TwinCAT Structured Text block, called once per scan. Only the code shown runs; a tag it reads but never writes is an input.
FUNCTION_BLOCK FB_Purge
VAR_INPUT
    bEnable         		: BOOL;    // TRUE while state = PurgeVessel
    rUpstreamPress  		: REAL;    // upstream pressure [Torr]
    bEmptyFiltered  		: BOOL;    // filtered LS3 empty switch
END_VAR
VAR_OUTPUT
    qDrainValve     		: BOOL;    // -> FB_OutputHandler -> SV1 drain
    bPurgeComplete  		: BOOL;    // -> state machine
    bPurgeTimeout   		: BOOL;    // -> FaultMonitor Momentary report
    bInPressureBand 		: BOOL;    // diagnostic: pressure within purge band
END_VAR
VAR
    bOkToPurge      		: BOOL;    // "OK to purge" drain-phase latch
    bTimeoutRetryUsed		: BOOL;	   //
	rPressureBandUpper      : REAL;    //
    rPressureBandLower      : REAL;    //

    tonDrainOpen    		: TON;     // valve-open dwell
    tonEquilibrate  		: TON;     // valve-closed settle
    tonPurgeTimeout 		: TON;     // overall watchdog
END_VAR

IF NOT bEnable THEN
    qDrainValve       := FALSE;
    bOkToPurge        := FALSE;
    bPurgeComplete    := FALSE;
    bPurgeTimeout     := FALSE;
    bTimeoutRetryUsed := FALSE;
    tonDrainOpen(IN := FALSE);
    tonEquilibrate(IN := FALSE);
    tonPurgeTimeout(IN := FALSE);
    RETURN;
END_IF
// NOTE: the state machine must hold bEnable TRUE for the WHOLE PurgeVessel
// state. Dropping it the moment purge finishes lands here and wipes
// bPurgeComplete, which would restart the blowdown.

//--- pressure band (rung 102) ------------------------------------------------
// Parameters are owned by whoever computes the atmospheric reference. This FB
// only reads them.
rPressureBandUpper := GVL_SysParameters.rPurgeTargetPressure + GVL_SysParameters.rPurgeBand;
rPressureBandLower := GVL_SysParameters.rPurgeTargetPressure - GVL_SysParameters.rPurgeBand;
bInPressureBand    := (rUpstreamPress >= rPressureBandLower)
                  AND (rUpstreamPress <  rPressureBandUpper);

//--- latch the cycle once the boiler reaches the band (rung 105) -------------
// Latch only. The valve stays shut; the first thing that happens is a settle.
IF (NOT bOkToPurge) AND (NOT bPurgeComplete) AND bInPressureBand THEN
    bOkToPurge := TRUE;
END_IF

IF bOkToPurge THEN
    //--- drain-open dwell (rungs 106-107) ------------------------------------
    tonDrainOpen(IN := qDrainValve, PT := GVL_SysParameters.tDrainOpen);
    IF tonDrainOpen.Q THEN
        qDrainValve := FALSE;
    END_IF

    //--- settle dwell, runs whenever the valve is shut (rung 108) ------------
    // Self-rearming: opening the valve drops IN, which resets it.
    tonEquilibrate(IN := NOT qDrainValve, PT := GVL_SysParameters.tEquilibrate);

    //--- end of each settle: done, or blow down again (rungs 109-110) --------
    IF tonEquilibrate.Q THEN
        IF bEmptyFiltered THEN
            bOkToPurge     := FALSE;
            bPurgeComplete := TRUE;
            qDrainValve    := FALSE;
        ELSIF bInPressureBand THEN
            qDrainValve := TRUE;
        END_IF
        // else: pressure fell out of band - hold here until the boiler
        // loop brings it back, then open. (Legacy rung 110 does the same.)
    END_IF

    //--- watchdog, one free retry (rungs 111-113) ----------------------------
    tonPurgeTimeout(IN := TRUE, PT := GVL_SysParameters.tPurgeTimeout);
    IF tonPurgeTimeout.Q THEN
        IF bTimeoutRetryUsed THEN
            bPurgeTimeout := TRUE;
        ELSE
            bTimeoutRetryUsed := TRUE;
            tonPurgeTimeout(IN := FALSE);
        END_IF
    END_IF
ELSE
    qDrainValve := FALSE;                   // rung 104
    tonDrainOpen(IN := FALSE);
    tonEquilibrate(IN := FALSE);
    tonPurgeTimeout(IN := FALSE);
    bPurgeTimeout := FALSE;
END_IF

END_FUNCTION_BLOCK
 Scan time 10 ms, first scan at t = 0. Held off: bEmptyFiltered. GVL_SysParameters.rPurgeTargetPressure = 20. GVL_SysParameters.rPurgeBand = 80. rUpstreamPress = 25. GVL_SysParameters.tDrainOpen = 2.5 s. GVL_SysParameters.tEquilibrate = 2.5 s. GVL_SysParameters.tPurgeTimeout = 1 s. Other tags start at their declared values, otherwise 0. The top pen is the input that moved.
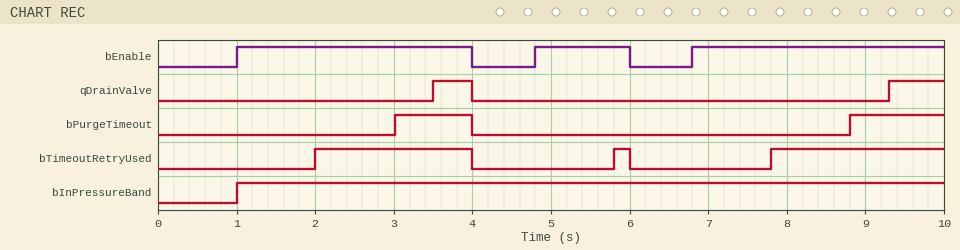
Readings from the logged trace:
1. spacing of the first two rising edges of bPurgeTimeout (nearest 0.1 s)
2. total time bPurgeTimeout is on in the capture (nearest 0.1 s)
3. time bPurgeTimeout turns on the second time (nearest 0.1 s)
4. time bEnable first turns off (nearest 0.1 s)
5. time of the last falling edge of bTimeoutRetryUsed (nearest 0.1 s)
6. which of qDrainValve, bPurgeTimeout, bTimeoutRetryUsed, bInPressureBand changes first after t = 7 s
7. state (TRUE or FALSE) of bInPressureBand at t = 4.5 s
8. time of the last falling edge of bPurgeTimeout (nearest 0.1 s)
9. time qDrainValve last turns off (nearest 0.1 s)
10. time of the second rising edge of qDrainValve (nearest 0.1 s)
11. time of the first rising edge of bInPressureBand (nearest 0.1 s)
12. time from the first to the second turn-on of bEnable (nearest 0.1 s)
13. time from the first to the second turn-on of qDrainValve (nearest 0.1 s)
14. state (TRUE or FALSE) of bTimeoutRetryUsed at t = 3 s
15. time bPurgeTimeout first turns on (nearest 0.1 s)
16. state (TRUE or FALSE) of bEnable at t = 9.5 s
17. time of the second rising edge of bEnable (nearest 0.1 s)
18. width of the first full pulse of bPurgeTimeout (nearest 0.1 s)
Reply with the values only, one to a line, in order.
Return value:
5.8 s
2.2 s
8.8 s
4.0 s
6.0 s
bTimeoutRetryUsed
TRUE
4.0 s
4.0 s
9.3 s
1.0 s
3.8 s
5.8 s
TRUE
3.0 s
TRUE
4.8 s
1.0 s
